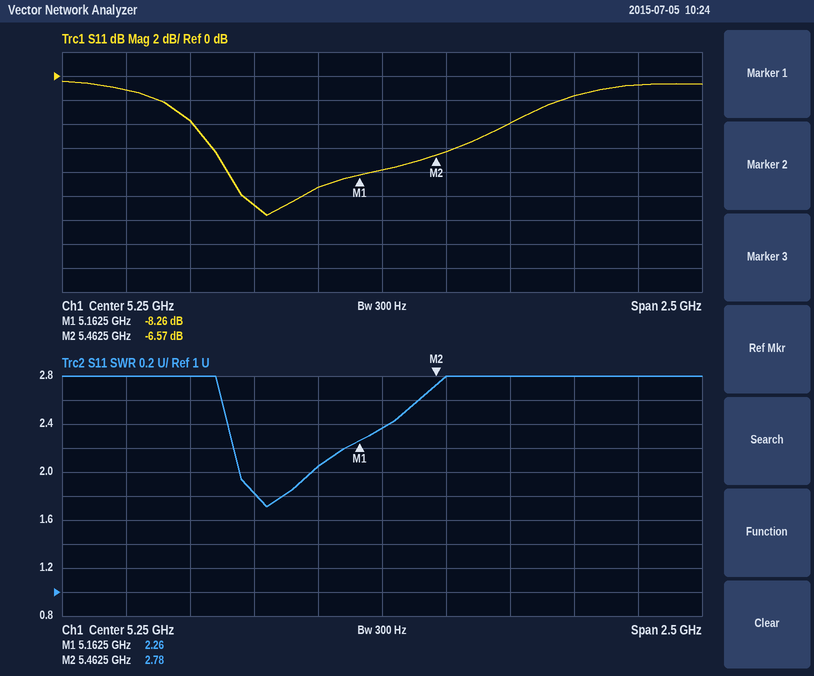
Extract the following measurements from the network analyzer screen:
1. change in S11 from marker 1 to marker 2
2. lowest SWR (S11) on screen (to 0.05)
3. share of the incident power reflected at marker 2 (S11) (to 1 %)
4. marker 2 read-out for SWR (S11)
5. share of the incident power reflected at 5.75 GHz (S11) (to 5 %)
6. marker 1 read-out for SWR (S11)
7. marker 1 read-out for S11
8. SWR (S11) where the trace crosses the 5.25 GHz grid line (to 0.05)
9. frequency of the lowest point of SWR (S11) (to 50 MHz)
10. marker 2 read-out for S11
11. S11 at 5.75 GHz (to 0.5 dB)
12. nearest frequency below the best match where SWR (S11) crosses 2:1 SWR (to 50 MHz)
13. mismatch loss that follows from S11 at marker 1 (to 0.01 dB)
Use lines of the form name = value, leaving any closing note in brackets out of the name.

change in S11 from marker 1 to marker 2 = 1.69 dB
lowest SWR (S11) on screen = 1.70
share of the incident power reflected at marker 2 (S11) = 22 %
marker 2 read-out for SWR = 2.78
share of the incident power reflected at 5.75 GHz (S11) = 40 %
marker 1 read-out for SWR = 2.26
marker 1 read-out for S11 = -8.26 dB
SWR (S11) where the trace crosses the 5.25 GHz grid line = 2.35
frequency of the lowest point of SWR (S11) = 4.80 GHz
marker 2 read-out for S11 = -6.57 dB
S11 at 5.75 GHz = -4.0 dB
nearest frequency below the best match where SWR (S11) crosses 2:1 SWR = 4.70 GHz
mismatch loss that follows from S11 at marker 1 = 0.70 dB
